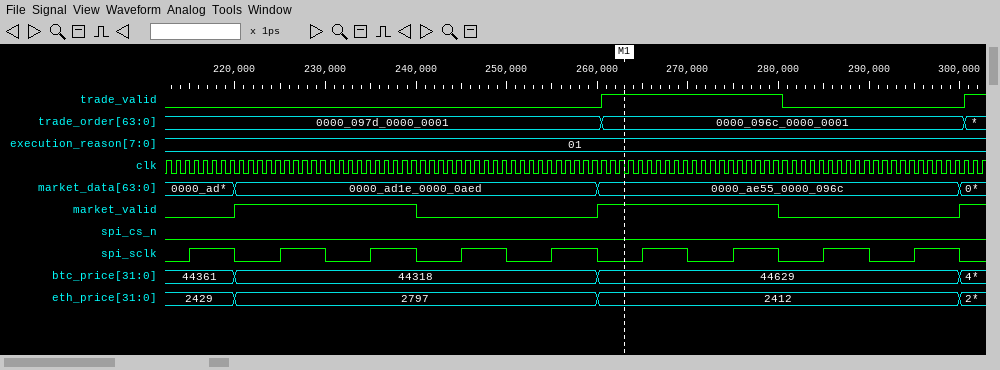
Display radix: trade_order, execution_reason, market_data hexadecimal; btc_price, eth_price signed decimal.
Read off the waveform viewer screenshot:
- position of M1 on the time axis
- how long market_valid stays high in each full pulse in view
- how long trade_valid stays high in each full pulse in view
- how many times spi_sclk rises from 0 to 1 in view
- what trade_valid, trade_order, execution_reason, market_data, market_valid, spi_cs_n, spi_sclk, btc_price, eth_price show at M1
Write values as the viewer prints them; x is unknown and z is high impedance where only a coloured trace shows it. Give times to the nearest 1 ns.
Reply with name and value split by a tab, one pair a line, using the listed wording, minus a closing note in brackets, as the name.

position of M1 on the time axis	263 ns
how long market_valid stays high in each full pulse in view	20 ns, 20 ns
how long trade_valid stays high in each full pulse in view	20 ns
how many times spi_sclk rises from 0 to 1 in view	9
what trade_valid, trade_order, execution_reason, market_data, market_valid, spi_cs_n, spi_sclk, btc_price, eth_price show at M1	trade_valid=1, trade_order=0000_096c_0000_0001, execution_reason=01, market_data=0000_ae55_0000_096c, market_valid=1, spi_cs_n=0, spi_sclk=0, btc_price=44629, eth_price=2412
